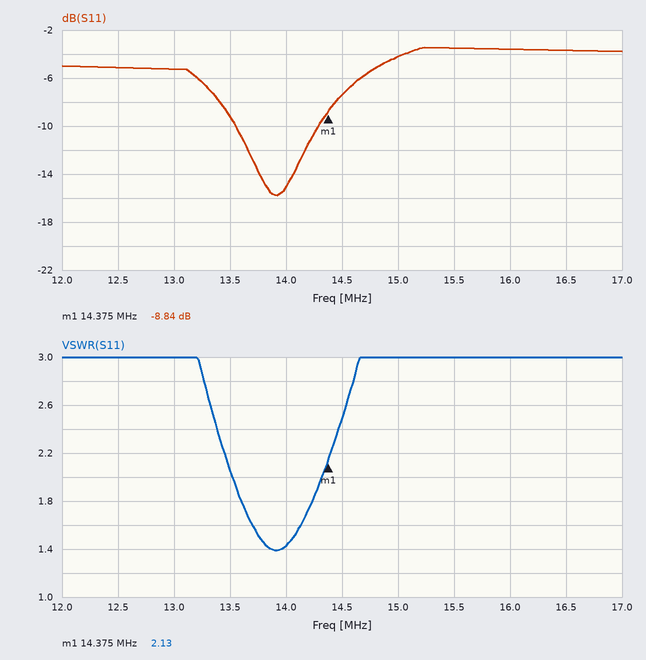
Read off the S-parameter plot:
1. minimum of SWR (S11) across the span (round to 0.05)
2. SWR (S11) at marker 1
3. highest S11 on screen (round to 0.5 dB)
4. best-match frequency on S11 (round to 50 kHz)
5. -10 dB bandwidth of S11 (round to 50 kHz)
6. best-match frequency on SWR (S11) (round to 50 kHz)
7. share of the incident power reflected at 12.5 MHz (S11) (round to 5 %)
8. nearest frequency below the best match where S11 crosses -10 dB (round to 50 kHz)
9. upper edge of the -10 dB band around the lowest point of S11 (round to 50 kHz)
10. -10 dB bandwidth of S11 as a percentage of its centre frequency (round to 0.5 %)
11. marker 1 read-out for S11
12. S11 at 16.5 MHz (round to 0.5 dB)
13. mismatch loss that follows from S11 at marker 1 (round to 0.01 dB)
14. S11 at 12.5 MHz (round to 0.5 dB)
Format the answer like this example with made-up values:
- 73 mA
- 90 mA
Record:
- 1.40
- 2.13
- -3.5 dB
- 13.90 MHz
- 750 kHz
- 13.90 MHz
- 30 %
- 13.55 MHz
- 14.30 MHz
- 5.5 %
- -8.84 dB
- -3.5 dB
- 0.61 dB
- -5.0 dB
